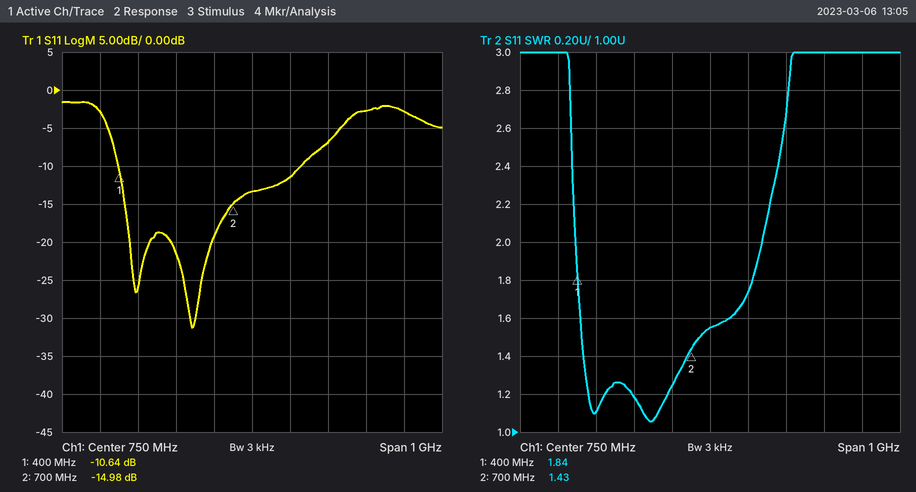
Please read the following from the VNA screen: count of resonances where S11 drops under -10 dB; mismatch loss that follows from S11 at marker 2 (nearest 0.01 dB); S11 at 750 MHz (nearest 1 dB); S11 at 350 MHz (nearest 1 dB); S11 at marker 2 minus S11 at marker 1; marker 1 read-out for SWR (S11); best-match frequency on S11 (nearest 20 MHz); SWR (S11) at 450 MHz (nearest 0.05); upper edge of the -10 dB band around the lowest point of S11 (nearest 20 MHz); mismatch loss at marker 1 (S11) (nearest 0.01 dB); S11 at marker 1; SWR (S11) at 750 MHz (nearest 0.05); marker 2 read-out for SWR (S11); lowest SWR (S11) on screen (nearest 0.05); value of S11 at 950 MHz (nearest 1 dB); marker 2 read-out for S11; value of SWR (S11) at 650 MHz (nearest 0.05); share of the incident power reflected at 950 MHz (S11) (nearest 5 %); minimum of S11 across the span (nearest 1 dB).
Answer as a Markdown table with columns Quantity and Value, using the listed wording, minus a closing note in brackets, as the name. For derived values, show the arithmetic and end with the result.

| Quantity | Value |
|---|---|
| count of resonances where S11 drops under -10 dB | 2 |
| mismatch loss that follows from S11 at marker 2 | −10 log10(1 − 10^(-14.98/10)) ≈ 0.14 dB |
| S11 at 750 MHz | -13 dB |
| S11 at 350 MHz | -3 dB |
| S11 at marker 2 minus S11 at marker 1 | -14.98 − (-10.64) = -4.34 dB |
| marker 1 read-out for SWR | 1.84 |
| best-match frequency on S11 | 600 MHz |
| SWR (S11) at 450 MHz | 1.10 |
| upper edge of the -10 dB band around the lowest point of S11 | 880 MHz |
| mismatch loss at marker 1 (S11) | −10 log10(1 − 10^(-10.64/10)) ≈ 0.39 dB |
| S11 at marker 1 | -10.64 dB |
| SWR (S11) at 750 MHz | 1.55 |
| marker 2 read-out for SWR | 1.43 |
| lowest SWR (S11) on screen | 1.05 |
| value of S11 at 950 MHz | -7 dB |
| marker 2 read-out for S11 | -14.98 dB |
| value of SWR (S11) at 650 MHz | 1.25 |
| share of the incident power reflected at 950 MHz (S11) | 10^(-7/10) ≈ 20 % |
| minimum of S11 across the span | -31 dB |
